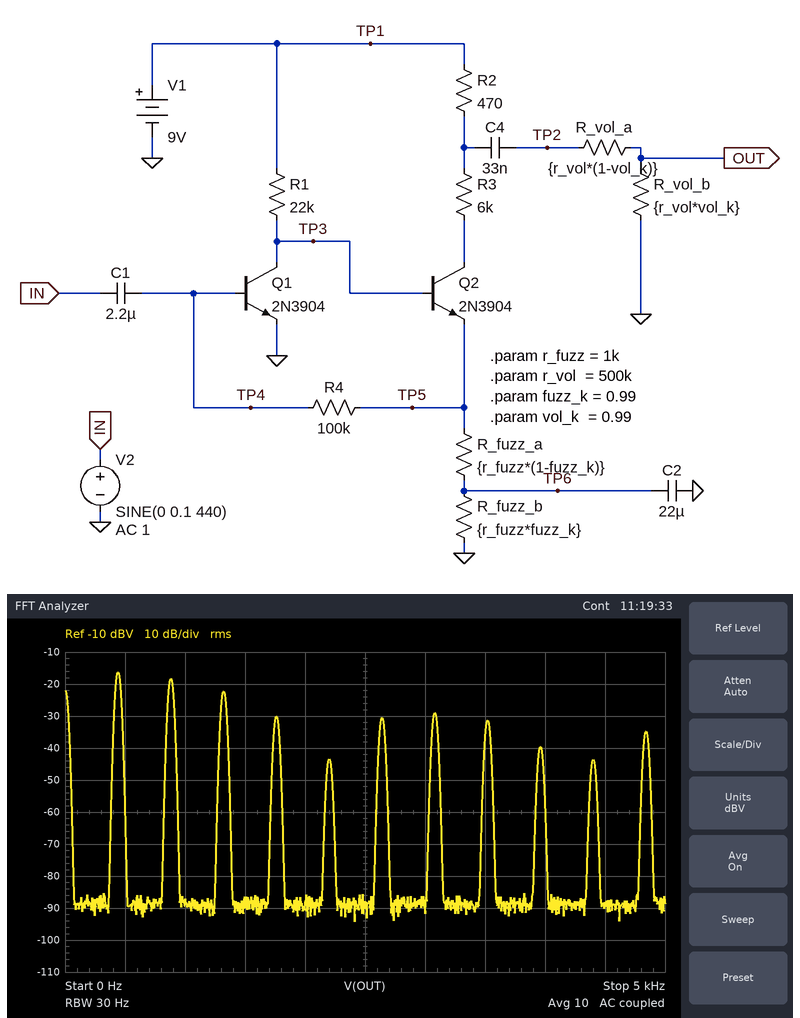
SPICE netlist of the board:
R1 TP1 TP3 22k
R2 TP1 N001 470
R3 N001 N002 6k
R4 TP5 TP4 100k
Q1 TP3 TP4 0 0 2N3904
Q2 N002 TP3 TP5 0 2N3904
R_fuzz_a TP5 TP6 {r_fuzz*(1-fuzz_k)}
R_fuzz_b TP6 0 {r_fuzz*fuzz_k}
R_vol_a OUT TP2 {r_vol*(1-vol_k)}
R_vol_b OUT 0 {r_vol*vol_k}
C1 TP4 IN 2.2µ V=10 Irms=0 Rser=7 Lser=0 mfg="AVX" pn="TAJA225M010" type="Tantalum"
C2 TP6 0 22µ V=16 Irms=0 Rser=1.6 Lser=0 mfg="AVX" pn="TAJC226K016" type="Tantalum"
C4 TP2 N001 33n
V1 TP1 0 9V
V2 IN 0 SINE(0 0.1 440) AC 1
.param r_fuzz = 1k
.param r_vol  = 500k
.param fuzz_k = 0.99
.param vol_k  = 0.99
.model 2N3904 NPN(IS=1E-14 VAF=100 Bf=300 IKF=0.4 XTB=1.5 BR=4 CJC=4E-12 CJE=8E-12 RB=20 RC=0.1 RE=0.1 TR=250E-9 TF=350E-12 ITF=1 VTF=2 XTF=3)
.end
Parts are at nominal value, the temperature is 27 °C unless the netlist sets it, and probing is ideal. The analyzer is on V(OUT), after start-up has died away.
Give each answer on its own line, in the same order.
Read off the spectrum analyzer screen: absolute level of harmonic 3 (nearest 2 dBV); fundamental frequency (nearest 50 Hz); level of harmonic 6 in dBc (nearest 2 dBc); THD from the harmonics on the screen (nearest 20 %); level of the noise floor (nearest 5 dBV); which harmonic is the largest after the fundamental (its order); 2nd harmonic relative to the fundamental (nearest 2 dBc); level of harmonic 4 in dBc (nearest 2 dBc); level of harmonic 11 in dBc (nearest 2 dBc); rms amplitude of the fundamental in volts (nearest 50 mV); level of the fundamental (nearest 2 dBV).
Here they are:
-22 dBV
450 Hz
-14 dBc
100 %
-90 dBV
2
-2 dBc
-14 dBc
-18 dBc
150 mV
-16 dBV
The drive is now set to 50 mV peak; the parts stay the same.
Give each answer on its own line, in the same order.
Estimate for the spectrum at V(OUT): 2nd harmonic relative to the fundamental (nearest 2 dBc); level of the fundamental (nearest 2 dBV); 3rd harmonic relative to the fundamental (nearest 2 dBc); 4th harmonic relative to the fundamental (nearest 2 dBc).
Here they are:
-4 dBc
-14 dBV
-10 dBc
-28 dBc
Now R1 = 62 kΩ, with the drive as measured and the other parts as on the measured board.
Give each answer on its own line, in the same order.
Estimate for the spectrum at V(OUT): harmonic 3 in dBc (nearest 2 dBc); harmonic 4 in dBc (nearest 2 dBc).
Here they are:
-8 dBc
-28 dBc
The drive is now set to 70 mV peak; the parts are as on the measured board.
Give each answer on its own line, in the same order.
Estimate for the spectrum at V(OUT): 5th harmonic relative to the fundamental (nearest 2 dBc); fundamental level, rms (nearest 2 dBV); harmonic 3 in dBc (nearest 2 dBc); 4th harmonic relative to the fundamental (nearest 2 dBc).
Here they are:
-16 dBc
-16 dBV
-8 dBc
-22 dBc
